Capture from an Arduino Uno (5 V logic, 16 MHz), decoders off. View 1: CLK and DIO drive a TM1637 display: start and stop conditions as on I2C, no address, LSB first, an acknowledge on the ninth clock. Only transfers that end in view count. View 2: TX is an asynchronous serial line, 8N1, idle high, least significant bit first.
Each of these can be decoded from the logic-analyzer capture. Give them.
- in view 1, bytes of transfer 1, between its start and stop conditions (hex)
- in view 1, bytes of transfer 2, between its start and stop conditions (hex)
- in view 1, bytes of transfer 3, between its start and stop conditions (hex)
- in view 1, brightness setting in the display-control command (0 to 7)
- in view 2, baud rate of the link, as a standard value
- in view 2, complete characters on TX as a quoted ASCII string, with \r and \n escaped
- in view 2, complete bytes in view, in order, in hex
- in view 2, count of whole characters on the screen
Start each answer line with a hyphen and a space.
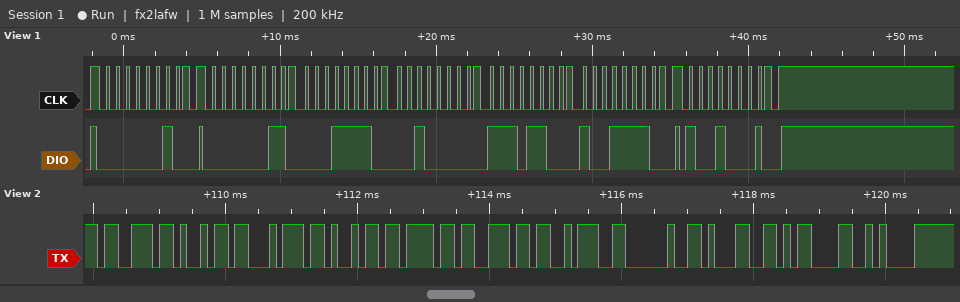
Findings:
- 40
- C0 78 04 37 79
- 89
- 1
- 9600 baud
- "sition: 1\r\n"
- 73 69 74 69 6F 6E 3A 20 31 0D 0A
- 11
